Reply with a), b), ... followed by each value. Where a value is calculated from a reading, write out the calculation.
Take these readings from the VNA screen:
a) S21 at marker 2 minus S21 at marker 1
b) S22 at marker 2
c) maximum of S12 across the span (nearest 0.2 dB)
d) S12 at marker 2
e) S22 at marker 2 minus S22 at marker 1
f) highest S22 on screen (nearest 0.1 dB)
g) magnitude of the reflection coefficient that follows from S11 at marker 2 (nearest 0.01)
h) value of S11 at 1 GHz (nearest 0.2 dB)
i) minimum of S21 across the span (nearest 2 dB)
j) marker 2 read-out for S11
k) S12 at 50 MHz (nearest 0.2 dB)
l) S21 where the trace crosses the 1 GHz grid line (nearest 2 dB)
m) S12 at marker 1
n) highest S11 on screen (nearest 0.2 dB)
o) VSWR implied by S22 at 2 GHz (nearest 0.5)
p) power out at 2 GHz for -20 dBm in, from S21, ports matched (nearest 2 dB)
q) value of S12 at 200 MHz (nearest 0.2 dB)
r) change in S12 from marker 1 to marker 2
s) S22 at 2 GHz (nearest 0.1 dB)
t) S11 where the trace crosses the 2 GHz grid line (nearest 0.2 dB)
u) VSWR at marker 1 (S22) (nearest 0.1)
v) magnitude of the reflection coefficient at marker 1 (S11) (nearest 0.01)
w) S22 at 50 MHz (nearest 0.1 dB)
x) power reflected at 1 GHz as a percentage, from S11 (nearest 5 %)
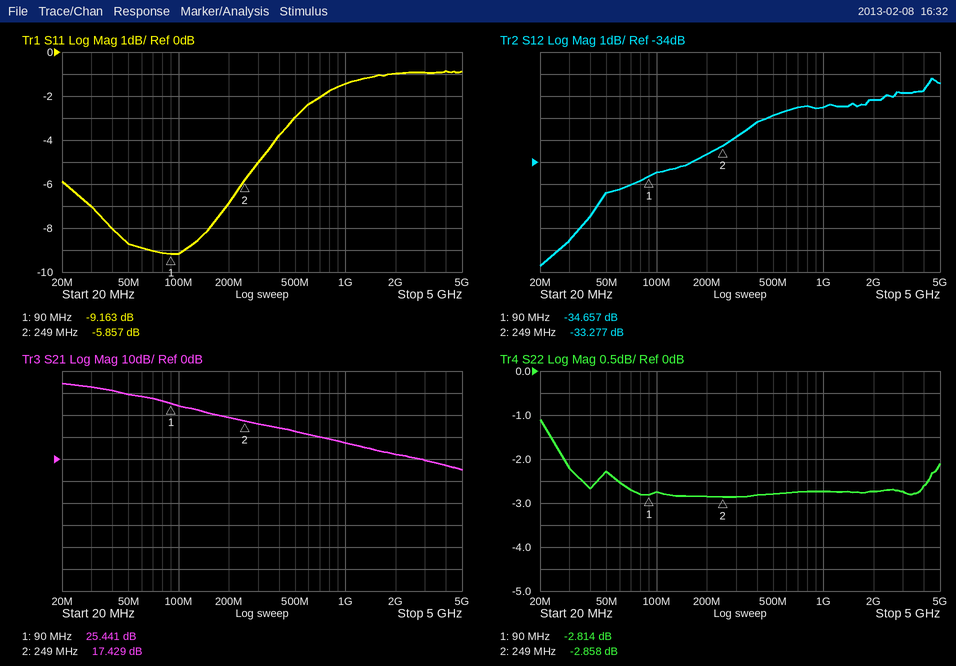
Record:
a) 17.429 − (25.441) = -8.012 dB
b) -2.858 dB
c) -30.2 dB
d) -33.277 dB
e) -2.858 − (-2.814) = -0.044 dB
f) -1.1 dB
g) 10^(-5.857/20) ≈ 0.51
h) -1.4 dB
i) -4 dB
j) -5.857 dB
k) -35.4 dB
l) 8 dB
m) -34.657 dB
n) -0.8 dB
o) |Γ| = 10^(-2.7/20) = 0.7328; VSWR = (1 + 0.7328)/(1 − 0.7328) ≈ 6.5
p) -20 dBm + (2 dB) = -18 dBm
q) -33.6 dB
r) -33.277 − (-34.657) = 1.380 dB
s) -2.7 dB
t) -1.0 dB
u) (1 + 0.7233)/(1 − 0.7233) ≈ 6.2
v) 10^(-9.163/20) ≈ 0.35
w) -2.3 dB
x) 10^(-1.4/10) ≈ 72.4 %, so 70 % to the nearest 5 %
